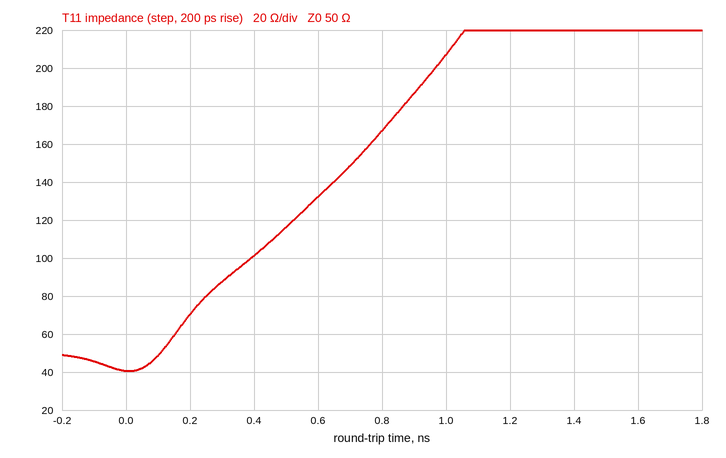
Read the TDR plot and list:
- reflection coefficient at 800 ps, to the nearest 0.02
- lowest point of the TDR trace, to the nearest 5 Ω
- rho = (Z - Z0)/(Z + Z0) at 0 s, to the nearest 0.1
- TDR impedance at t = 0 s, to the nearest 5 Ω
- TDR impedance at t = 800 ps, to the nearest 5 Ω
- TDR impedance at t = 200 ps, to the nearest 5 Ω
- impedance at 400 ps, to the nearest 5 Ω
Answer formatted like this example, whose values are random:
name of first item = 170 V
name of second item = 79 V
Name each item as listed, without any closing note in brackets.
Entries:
reflection coefficient at 800 ps, to the nearest 0.02 = +0.54
lowest point of the TDR trace, to the nearest 5 Ω = 40 Ω
rho = (Z - Z0)/(Z + Z0) at 0 s, to the nearest 0.1 = -0.1
TDR impedance at t = 0 s, to the nearest 5 Ω = 40 Ω
TDR impedance at t = 800 ps, to the nearest 5 Ω = 165 Ω
TDR impedance at t = 200 ps, to the nearest 5 Ω = 70 Ω
impedance at 400 ps, to the nearest 5 Ω = 100 Ω
